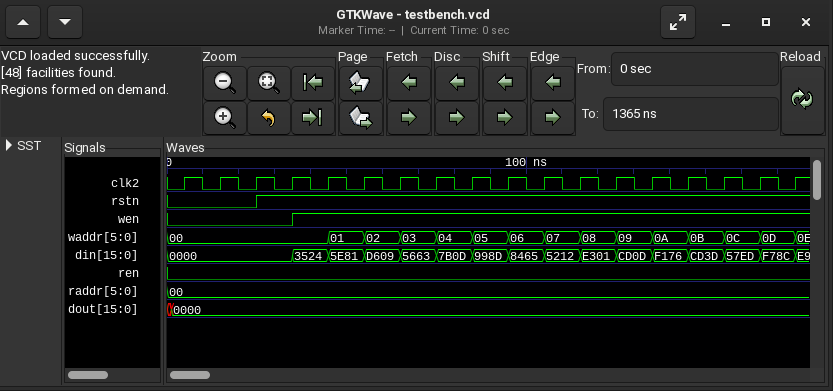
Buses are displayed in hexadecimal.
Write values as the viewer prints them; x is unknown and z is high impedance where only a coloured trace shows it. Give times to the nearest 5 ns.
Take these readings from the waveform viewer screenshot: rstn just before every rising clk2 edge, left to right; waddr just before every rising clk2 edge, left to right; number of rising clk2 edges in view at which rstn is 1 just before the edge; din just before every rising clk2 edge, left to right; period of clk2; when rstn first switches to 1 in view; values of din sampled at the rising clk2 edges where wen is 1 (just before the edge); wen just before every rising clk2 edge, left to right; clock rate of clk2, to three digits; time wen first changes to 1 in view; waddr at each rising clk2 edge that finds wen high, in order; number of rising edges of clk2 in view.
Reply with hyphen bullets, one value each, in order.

- 0 0 0 1 1 1 1 1 1 1 1 1 1 1 1 1 1 1
- 00, 00, 00, 00, 00, 01, 02, 03, 04, 05, 06, 07, 08, 09, 0A, 0B, 0C, 0D
- 15
- 0000, 0000, 0000, 0000, 3524, 5E81, D609, 5663, 7B0D, 998D, 8465, 5212, E301, CD0D, F176, CD3D, 57ED, F78C
- 10 ns
- 25 ns
- 3524, 5E81, D609, 5663, 7B0D, 998D, 8465, 5212, E301, CD0D, F176, CD3D, 57ED, F78C
- 0 0 0 0 1 1 1 1 1 1 1 1 1 1 1 1 1 1
- 100 MHz
- 35 ns
- 00, 01, 02, 03, 04, 05, 06, 07, 08, 09, 0A, 0B, 0C, 0D
- 18
